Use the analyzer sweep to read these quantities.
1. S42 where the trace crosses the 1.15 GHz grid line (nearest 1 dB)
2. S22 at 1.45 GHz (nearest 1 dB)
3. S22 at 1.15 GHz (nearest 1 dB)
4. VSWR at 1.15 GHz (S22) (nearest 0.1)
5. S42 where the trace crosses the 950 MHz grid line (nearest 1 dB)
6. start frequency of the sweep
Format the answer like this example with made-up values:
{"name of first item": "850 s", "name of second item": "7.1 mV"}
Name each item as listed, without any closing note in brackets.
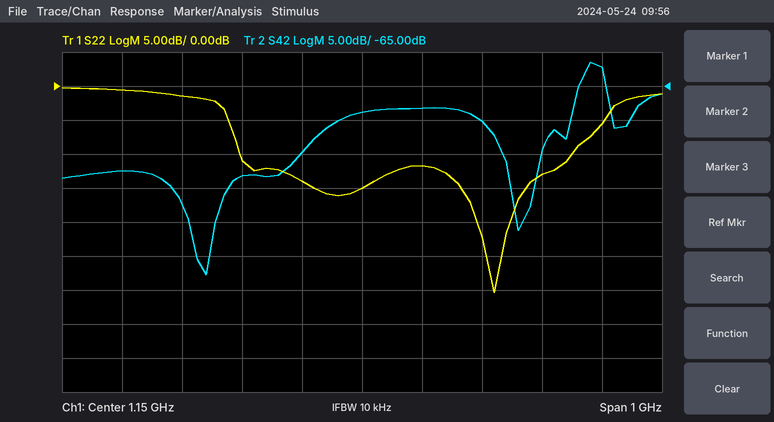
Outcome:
{"S42 where the trace crosses the 1.15 GHz grid line": "-69 dB", "S22 at 1.45 GHz": "-13 dB", "S22 at 1.15 GHz": "-15 dB", "VSWR at 1.15 GHz (S22)": "1.4", "S42 where the trace crosses the 950 MHz grid line": "-78 dB", "start frequency of the sweep": "650 MHz"}
